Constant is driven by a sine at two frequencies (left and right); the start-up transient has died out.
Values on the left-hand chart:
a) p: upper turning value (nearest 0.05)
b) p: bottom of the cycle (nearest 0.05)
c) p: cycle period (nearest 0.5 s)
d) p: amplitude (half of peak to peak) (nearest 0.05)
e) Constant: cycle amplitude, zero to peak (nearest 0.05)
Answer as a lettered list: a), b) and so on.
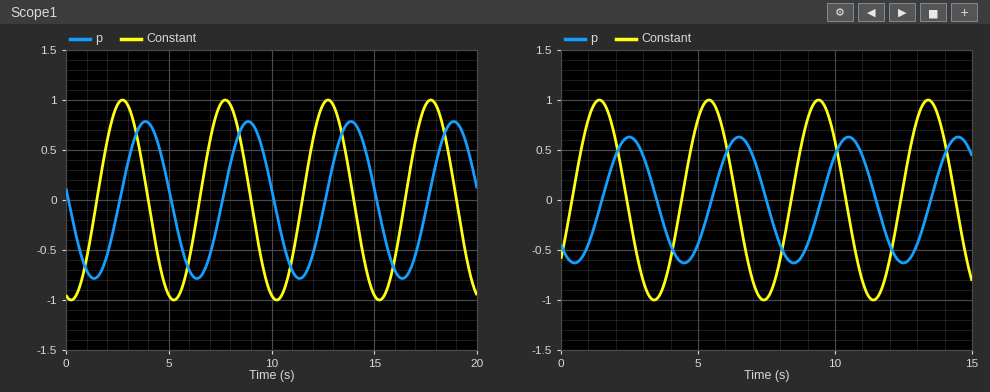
a) 0.80
b) -0.80
c) 5.0 s
d) 0.80
e) 1.00
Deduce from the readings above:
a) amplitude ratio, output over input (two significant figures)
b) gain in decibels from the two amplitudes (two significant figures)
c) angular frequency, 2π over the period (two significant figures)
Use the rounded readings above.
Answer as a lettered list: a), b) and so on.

a) 0.80
b) -1.9 dB
c) 1.3 rad/s
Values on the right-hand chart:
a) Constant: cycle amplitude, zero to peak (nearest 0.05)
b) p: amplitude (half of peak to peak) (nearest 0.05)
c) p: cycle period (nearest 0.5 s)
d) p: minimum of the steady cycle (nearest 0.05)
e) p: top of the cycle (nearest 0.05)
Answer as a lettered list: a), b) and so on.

a) 1.00
b) 0.65
c) 4.0 s
d) -0.65
e) 0.65
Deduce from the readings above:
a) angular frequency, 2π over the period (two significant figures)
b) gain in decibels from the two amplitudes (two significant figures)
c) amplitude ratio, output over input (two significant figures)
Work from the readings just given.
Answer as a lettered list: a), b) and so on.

a) 1.6 rad/s
b) -3.7 dB
c) 0.65
